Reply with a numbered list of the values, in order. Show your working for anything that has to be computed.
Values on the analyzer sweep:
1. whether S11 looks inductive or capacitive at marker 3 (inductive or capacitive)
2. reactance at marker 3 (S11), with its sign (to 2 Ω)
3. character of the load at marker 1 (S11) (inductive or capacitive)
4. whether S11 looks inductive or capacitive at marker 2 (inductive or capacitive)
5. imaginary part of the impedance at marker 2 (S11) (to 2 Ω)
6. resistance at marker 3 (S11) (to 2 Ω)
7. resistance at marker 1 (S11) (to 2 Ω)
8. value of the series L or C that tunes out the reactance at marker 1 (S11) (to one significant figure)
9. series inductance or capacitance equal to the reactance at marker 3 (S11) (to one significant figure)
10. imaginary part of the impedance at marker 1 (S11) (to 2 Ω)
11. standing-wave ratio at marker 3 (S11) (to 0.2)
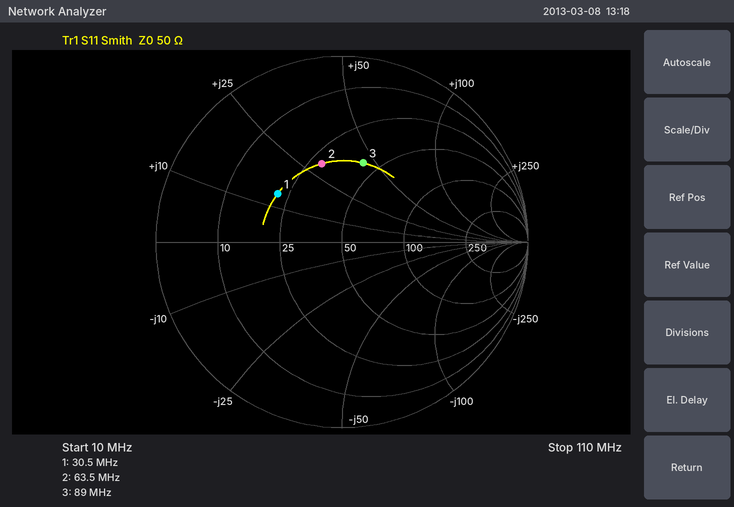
1. inductive
2. +44 Ω
3. inductive
4. inductive
5. +30 Ω
6. 42 Ω
7. 22 Ω
8. C = 1/(2π × 30.5 MHz × 14 Ω) ≈ 373 pF, so 400 pF to one significant figure
9. L = 44 Ω/(2π × 89 MHz) ≈ 78.7 nH, so 80 nH to one significant figure
10. +14 Ω
11. 2.6
